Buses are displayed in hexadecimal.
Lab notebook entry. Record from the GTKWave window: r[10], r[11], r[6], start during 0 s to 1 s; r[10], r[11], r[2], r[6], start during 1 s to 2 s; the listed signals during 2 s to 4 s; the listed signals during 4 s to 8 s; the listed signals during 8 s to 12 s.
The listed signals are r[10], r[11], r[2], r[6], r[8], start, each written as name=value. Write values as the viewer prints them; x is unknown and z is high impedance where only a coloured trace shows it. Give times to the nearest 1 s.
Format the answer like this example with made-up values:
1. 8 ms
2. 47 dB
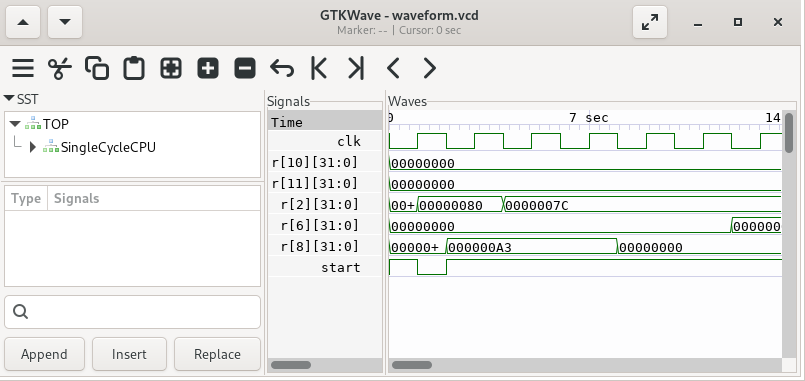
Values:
1. r[10]=00000000, r[11]=00000000, r[6]=00000000, start=1
2. r[10]=00000000, r[11]=00000000, r[2]=00000080, r[6]=00000000, start=0
3. r[10]=00000000, r[11]=00000000, r[2]=00000080, r[6]=00000000, r[8]=000000A3, start=1
4. r[10]=00000000, r[11]=00000000, r[2]=0000007C, r[6]=00000000, r[8]=000000A3, start=1
5. r[10]=00000000, r[11]=00000000, r[2]=0000007C, r[6]=00000000, r[8]=00000000, start=1
